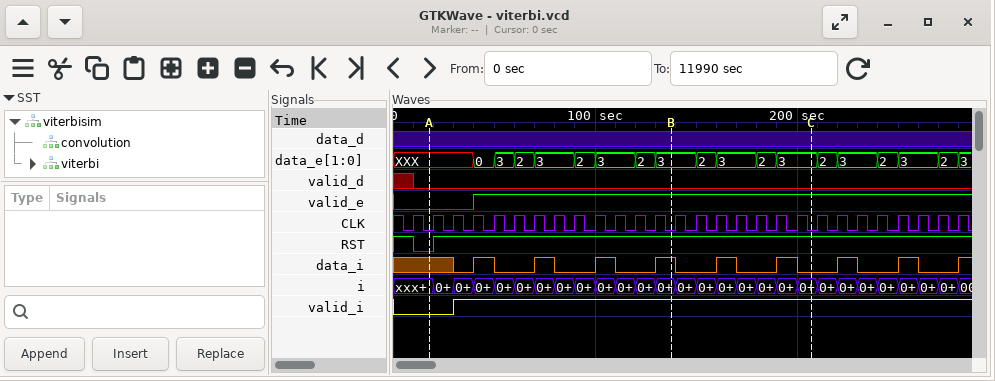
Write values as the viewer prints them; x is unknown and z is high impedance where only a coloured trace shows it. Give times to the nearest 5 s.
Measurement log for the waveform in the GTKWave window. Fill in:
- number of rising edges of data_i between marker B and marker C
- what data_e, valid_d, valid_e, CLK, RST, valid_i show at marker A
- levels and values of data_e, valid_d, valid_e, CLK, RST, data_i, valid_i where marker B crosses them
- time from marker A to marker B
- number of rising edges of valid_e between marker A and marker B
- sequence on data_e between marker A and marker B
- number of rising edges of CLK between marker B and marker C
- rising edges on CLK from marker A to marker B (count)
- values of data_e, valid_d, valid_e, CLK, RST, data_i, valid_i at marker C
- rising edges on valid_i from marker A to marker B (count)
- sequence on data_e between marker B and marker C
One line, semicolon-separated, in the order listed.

2; data_e=XXX, valid_d=0, valid_e=0, CLK=0, RST=0, valid_i=0; data_e=3, valid_d=0, valid_e=1, CLK=0, RST=1, data_i=1, valid_i=1; 120 s; 1; XXX, 0, 3, 2, 3, 2, 3, 2, 3; 7; 12; data_e=3, valid_d=0, valid_e=1, CLK=0, RST=1, data_i=0, valid_i=1; 1; 3, 2, 3, 2, 3
